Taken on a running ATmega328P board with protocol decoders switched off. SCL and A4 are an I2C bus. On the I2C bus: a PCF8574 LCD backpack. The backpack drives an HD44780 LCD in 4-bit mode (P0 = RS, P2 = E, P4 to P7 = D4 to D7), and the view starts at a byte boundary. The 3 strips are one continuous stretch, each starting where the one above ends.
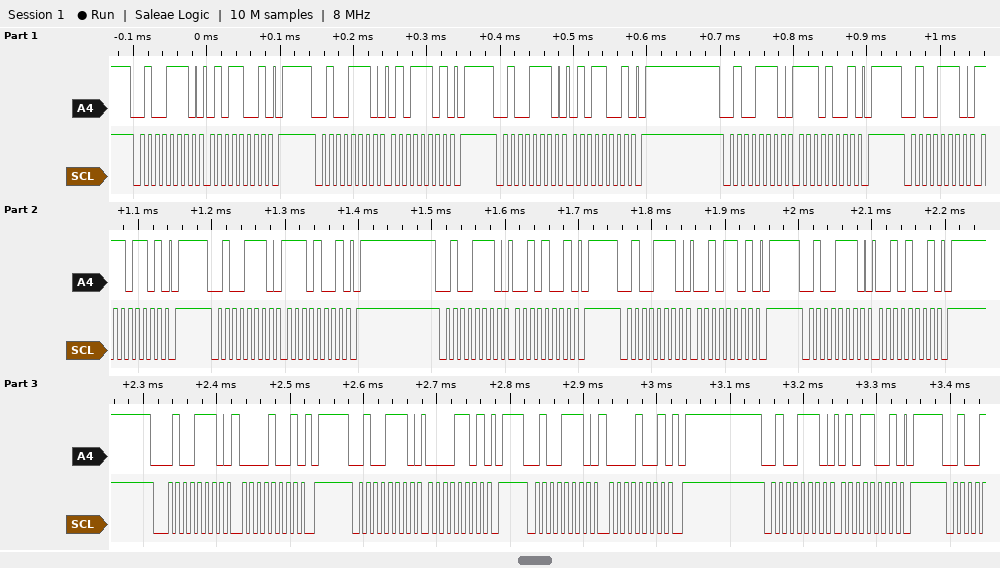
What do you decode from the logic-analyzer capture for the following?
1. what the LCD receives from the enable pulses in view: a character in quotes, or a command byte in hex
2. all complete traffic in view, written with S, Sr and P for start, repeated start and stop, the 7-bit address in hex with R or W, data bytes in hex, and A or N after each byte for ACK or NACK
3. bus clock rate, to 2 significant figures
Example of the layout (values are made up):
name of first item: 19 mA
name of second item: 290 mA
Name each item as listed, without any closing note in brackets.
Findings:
what the LCD receives from the enable pulses in view: a character in quotes, or a command byte in hex: '^' ' '
all complete traffic in view, written with S, Sr and P for start, repeated start and stop, the 7-bit address in hex with R or W, data bytes in hex, and A or N after each byte for ACK or NACK: S 27W A 59 A P S 27W A 5D A P S 27W A 59 A P S 27W A E9 A P S 27W A ED A P S 27W A E9 A P S 27W A 29 A P S 27W A 2D A P S 27W A 29 A P S 27W A 09 A P S 27W A 0D A P S 27W A 09 A P S 27W A 59 A P
bus clock rate, to 2 significant figures: 100 kHz
